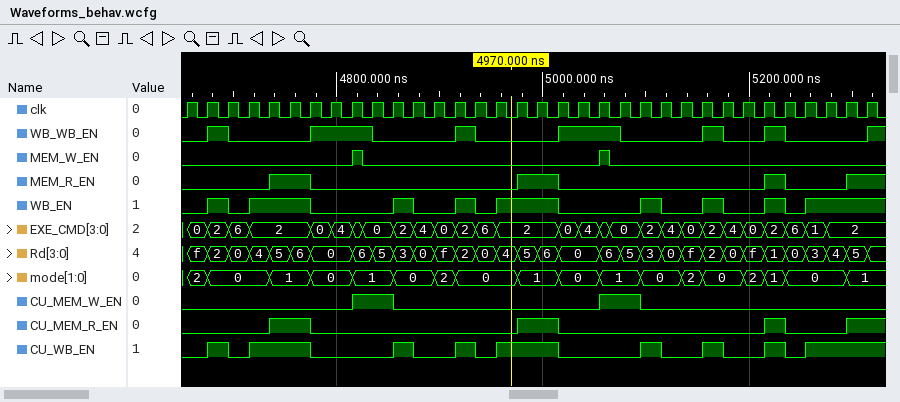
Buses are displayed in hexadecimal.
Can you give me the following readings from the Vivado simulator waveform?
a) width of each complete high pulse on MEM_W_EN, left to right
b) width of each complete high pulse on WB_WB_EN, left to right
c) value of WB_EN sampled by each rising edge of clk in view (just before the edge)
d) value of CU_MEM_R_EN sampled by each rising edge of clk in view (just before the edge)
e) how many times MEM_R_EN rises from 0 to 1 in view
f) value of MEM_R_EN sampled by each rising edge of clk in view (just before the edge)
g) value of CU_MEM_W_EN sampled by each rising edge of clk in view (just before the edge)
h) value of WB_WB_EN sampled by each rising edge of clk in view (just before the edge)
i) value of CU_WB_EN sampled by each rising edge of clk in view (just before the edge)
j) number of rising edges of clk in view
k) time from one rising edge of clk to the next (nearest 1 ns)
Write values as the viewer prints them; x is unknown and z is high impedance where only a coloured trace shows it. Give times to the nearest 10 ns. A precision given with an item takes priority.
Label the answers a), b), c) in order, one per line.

a) 10 ns, 10 ns
b) 20 ns, 60 ns, 20 ns, 60 ns, 20 ns, 20 ns
c) 0 0 1 0 1 1 1 0 0 0 0 1 0 0 1 0 1 1 1 0 0 0 0 1 0 0 1 0 0 1 0 1 1 1
d) 0 0 0 0 0 1 1 0 0 0 0 0 0 0 0 0 0 1 1 0 0 0 0 0 0 0 0 0 0 1 0 0 0 1
e) 4
f) 0 0 0 0 0 1 1 0 0 0 0 0 0 0 0 0 0 1 1 0 0 0 0 0 0 0 0 0 0 1 0 0 0 1
g) 0 0 0 0 0 0 0 0 0 1 1 0 0 0 0 0 0 0 0 0 0 1 1 0 0 0 0 0 0 0 0 0 0 0
h) 0 0 1 0 0 0 0 1 1 1 0 0 0 0 1 0 0 0 0 1 1 1 0 0 0 0 1 0 0 1 0 0 0 0
i) 0 0 1 0 1 1 1 0 0 0 0 1 0 0 1 0 1 1 1 0 0 0 0 1 0 0 1 0 0 1 0 1 1 1
j) 34
k) 20 ns
